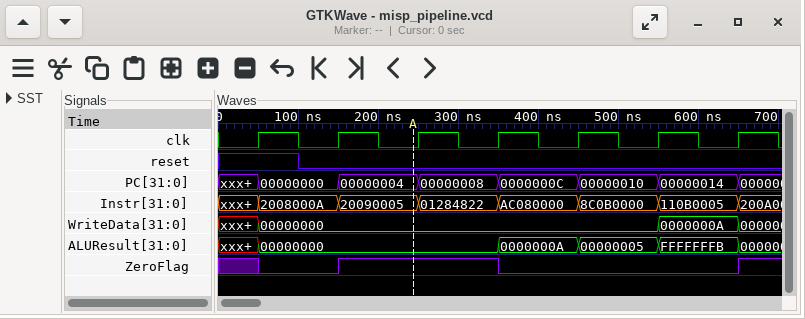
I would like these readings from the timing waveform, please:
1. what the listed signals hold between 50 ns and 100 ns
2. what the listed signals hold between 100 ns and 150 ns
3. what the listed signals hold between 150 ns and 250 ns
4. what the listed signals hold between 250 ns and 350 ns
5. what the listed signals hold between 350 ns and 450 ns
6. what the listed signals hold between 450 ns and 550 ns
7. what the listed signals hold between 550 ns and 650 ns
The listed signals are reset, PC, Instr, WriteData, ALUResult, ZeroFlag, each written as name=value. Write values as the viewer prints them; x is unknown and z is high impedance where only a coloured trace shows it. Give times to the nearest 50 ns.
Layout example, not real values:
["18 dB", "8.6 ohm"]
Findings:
["reset=1, PC=00000000, Instr=2008000A, WriteData=00000000, ALUResult=00000000, ZeroFlag=0", "reset=0, PC=00000000, Instr=2008000A, WriteData=00000000, ALUResult=00000000, ZeroFlag=0", "reset=0, PC=00000004, Instr=20090005, WriteData=00000000, ALUResult=00000000, ZeroFlag=1", "reset=0, PC=00000008, Instr=01284822, WriteData=00000000, ALUResult=00000000, ZeroFlag=1", "reset=0, PC=0000000C, Instr=AC080000, WriteData=00000000, ALUResult=0000000A, ZeroFlag=0", "reset=0, PC=00000010, Instr=8C0B0000, WriteData=00000000, ALUResult=00000005, ZeroFlag=0", "reset=0, PC=00000014, Instr=110B0005, WriteData=0000000A, ALUResult=FFFFFFFB, ZeroFlag=0"]
